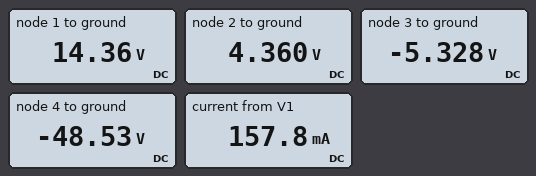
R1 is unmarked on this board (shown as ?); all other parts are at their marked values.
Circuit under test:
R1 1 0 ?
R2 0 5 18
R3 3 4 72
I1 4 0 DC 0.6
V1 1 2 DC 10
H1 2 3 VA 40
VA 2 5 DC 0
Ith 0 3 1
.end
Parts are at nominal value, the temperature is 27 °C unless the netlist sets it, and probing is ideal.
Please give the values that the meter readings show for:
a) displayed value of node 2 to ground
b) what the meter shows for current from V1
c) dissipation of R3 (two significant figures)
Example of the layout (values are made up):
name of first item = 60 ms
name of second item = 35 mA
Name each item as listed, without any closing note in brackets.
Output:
displayed value of node 2 to ground = 4.360 V
what the meter shows for current from V1 = 157.8 mA
dissipation of R3 = 26 W
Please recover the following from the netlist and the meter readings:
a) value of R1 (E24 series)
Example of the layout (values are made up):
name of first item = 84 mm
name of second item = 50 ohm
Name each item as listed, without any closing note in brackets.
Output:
value of R1 = 91 Ω
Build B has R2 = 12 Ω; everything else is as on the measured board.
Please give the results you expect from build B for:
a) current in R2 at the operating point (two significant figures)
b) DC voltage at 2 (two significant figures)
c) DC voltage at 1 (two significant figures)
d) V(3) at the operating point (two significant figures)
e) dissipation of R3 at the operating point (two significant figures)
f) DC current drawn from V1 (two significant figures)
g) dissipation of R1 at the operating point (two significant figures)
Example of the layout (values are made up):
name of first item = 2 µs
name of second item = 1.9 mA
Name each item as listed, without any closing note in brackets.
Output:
current in R2 at the operating point = 260 mA
DC voltage at 2 = 3.1 V
DC voltage at 1 = 13 V
V(3) at the operating point = -7.2 V
dissipation of R3 at the operating point = 26 W
DC current drawn from V1 = 140 mA
dissipation of R1 at the operating point = 1.9 W
